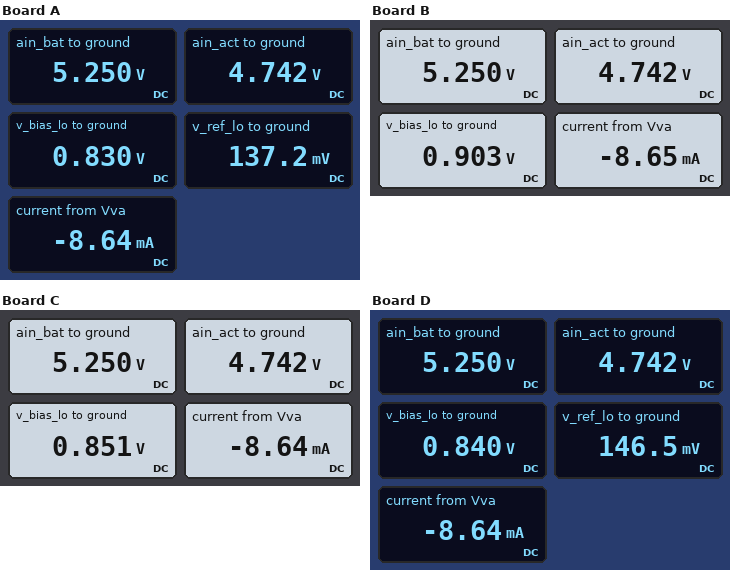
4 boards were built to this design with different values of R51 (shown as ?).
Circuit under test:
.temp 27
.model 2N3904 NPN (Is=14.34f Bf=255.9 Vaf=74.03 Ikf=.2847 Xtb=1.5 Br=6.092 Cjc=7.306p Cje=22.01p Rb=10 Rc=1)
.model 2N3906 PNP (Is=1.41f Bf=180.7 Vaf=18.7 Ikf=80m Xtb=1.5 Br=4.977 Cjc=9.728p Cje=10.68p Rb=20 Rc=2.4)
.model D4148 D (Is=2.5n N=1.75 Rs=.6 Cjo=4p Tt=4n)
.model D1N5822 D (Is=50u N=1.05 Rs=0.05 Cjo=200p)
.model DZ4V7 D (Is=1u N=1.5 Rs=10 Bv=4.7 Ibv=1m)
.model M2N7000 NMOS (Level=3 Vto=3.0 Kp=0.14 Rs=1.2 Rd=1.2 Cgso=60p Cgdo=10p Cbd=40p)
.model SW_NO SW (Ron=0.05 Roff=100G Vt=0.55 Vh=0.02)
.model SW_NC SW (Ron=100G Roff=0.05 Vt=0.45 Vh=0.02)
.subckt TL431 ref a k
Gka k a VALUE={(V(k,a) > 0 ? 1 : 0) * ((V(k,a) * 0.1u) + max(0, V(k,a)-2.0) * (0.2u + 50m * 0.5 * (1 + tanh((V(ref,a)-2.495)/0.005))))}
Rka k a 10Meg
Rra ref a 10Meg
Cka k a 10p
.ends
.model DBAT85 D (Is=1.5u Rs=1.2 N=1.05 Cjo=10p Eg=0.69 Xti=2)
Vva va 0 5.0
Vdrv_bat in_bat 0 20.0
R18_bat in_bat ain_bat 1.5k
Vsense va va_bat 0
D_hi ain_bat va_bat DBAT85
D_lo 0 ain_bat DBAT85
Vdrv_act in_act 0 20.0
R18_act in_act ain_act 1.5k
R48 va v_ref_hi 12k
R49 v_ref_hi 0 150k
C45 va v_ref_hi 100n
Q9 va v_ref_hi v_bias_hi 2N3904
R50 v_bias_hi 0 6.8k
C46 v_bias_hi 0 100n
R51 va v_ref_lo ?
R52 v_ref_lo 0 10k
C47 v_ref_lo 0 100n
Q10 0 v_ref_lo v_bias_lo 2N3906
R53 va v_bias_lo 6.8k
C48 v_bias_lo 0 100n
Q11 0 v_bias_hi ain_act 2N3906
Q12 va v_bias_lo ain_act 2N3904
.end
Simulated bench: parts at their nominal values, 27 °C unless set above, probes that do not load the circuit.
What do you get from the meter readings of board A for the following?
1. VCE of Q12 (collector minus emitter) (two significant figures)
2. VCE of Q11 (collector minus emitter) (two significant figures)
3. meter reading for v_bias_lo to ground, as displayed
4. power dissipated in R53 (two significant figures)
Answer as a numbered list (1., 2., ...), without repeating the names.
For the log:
1. 260 mV
2. -4.7 V
3. 0.830 V
4. 2.6 mW
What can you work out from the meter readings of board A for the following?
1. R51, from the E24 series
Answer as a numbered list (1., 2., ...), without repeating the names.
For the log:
1. 470 kΩ
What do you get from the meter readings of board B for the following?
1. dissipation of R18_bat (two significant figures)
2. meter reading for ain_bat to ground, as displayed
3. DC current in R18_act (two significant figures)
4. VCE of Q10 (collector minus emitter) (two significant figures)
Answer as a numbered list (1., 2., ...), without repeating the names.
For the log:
1. 150 mW
2. 5.250 V
3. 10 mA
4. -900 mV
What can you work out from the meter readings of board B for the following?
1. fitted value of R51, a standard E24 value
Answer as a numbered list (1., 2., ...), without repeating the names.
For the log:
1. 270 kΩ
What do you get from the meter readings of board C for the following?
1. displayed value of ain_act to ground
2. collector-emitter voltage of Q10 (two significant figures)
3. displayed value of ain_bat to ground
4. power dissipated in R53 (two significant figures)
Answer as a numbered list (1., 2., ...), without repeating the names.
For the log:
1. 4.742 V
2. -850 mV
3. 5.250 V
4. 2.5 mW
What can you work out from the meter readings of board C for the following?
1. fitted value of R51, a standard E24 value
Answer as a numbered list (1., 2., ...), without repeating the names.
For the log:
1. 390 kΩ
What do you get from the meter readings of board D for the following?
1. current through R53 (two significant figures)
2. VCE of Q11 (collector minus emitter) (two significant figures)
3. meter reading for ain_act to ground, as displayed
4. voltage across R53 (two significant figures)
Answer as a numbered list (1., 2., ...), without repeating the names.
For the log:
1. 610 µA
2. -4.7 V
3. 4.742 V
4. 4.2 V
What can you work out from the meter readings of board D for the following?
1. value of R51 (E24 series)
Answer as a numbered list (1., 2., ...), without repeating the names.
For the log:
1. 430 kΩ
